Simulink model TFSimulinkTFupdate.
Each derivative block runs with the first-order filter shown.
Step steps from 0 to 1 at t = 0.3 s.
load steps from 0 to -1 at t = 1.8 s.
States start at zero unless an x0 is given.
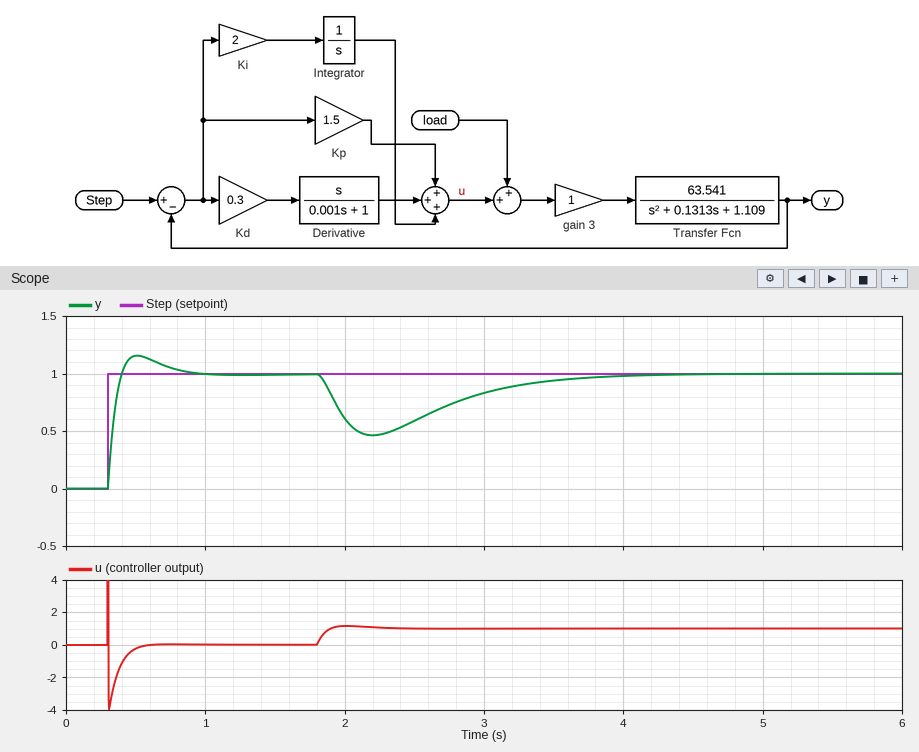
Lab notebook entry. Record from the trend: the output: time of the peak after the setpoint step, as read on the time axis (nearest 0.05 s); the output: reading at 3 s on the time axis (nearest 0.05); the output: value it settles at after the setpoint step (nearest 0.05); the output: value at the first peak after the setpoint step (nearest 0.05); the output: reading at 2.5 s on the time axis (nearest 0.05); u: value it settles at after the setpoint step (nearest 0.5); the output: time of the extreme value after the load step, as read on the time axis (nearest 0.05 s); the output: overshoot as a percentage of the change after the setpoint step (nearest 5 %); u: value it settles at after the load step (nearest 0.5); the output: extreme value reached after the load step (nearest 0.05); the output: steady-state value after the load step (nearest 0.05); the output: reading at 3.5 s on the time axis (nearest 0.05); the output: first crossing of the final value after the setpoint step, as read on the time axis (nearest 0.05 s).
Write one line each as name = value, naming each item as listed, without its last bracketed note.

the output: time of the peak after the setpoint step, as read on the time axis = 0.50 s
the output: reading at 3 s on the time axis = 0.85
the output: value it settles at after the setpoint step = 1.00
the output: value at the first peak after the setpoint step = 1.15
the output: reading at 2.5 s on the time axis = 0.60
u: value it settles at after the setpoint step = 0.0
the output: time of the extreme value after the load step, as read on the time axis = 2.20 s
the output: overshoot as a percentage of the change after the setpoint step = 15 %
u: value it settles at after the load step = 1.0
the output: extreme value reached after the load step = 0.45
the output: steady-state value after the load step = 1.00
the output: reading at 3.5 s on the time axis = 0.95
the output: first crossing of the final value after the setpoint step, as read on the time axis = 0.40 s
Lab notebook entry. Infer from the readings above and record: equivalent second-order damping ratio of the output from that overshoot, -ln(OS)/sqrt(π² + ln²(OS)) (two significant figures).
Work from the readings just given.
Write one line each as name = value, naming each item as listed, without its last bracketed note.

equivalent second-order damping ratio of the output from that overshoot, -ln(OS)/sqrt(π² + ln²(OS)) = 0.52
